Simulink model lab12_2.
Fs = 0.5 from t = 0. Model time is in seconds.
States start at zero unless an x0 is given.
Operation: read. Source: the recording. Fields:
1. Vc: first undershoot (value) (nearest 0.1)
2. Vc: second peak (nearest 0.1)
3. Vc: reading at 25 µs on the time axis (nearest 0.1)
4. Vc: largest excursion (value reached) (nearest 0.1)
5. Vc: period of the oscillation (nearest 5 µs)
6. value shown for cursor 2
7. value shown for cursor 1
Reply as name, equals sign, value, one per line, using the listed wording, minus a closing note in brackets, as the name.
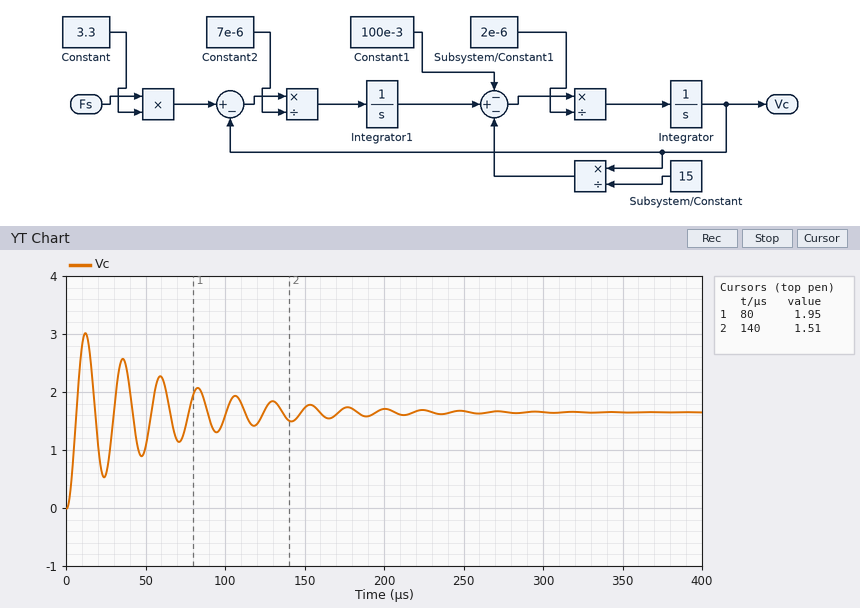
Vc: first undershoot (value) = 0.5
Vc: second peak = 2.6
Vc: reading at 25 µs on the time axis = 0.6
Vc: largest excursion (value reached) = 3.0
Vc: period of the oscillation = 25 µs
value shown for cursor 2 = 1.51
value shown for cursor 1 = 1.95
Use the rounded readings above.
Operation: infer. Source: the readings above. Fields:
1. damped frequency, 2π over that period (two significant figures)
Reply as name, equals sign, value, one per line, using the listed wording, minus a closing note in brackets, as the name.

damped frequency, 2π over that period = 0.25 rad/µs
